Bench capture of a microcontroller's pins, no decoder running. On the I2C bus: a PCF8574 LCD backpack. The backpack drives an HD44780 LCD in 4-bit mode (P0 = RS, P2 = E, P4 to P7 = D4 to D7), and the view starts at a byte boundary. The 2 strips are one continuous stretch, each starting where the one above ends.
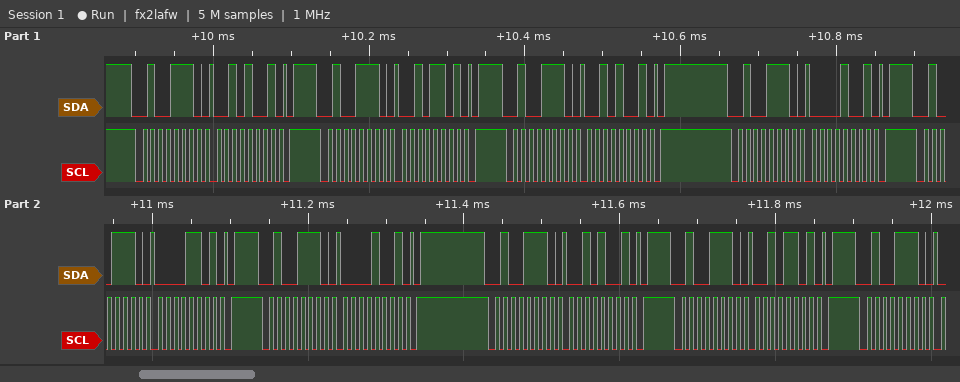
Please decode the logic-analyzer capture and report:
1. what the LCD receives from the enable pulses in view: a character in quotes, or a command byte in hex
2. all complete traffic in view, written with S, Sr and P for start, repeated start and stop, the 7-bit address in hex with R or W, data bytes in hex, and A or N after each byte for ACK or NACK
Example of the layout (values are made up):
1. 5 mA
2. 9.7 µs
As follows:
1. ' '
2. S 27W A 29 A P S 27W A 2D A P S 27W A 29 A P S 27W A 09 A P S 27W A 0D A P S 27W A 09 A P S 27W A 29 A P S 27W A 2D A P S 27W A
